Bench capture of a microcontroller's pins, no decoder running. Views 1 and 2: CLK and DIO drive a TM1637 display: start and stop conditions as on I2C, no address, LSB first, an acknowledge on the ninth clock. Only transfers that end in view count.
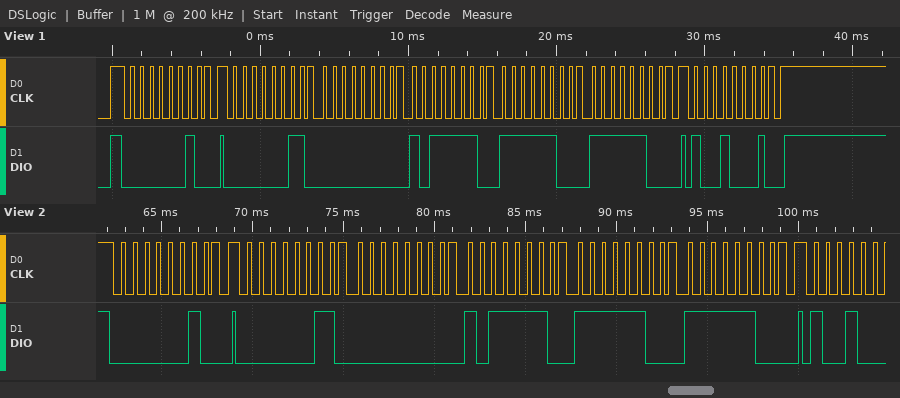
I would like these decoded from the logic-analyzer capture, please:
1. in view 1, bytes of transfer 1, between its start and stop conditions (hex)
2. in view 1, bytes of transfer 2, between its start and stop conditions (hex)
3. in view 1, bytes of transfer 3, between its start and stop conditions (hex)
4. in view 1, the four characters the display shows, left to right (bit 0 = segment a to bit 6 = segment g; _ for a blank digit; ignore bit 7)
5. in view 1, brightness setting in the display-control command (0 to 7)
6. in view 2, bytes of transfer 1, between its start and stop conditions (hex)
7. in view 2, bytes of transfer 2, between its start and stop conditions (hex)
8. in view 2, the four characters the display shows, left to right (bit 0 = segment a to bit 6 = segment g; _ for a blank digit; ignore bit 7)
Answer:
40
C0 00 7D 3F 3F
89
_600
1
40
C0 00 7D 3F 3F
_600
